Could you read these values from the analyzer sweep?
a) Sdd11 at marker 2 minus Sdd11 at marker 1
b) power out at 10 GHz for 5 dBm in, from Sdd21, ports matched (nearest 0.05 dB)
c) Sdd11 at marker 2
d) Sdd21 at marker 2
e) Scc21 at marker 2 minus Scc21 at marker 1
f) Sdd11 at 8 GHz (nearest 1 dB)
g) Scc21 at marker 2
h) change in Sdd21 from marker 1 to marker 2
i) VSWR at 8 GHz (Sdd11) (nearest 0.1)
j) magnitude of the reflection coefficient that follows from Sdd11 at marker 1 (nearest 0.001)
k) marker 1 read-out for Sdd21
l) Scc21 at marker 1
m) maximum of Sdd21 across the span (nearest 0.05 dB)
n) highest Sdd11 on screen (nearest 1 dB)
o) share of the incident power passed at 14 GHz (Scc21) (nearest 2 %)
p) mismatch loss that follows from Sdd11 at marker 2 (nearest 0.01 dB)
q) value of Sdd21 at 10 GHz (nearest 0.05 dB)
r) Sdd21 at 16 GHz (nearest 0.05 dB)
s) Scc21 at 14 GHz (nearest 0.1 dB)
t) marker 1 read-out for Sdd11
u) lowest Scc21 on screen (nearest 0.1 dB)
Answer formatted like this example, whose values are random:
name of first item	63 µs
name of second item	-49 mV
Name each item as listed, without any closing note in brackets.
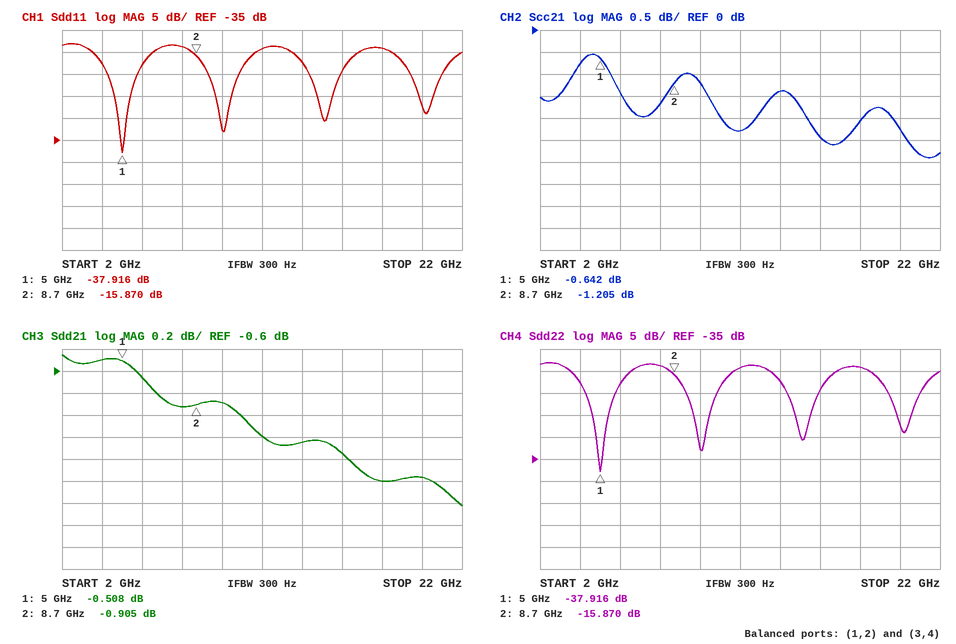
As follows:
Sdd11 at marker 2 minus Sdd11 at marker 1	22.046 dB
power out at 10 GHz for 5 dBm in, from Sdd21, ports matched	4.10 dBm
Sdd11 at marker 2	-15.870 dB
Sdd21 at marker 2	-0.905 dB
Scc21 at marker 2 minus Scc21 at marker 1	-0.563 dB
Sdd11 at 8 GHz	-14 dB
Scc21 at marker 2	-1.205 dB
change in Sdd21 from marker 1 to marker 2	-0.397 dB
VSWR at 8 GHz (Sdd11)	1.5
magnitude of the reflection coefficient that follows from Sdd11 at marker 1	0.013
marker 1 read-out for Sdd21	-0.508 dB
Scc21 at marker 1	-0.642 dB
maximum of Sdd21 across the span	-0.45 dB
highest Sdd11 on screen	-13 dB
share of the incident power passed at 14 GHz (Scc21)	72 %
mismatch loss that follows from Sdd11 at marker 2	0.11 dB
value of Sdd21 at 10 GHz	-0.90 dB
Sdd21 at 16 GHz	-1.35 dB
Scc21 at 14 GHz	-1.4 dB
marker 1 read-out for Sdd11	-37.916 dB
lowest Scc21 on screen	-2.9 dB
